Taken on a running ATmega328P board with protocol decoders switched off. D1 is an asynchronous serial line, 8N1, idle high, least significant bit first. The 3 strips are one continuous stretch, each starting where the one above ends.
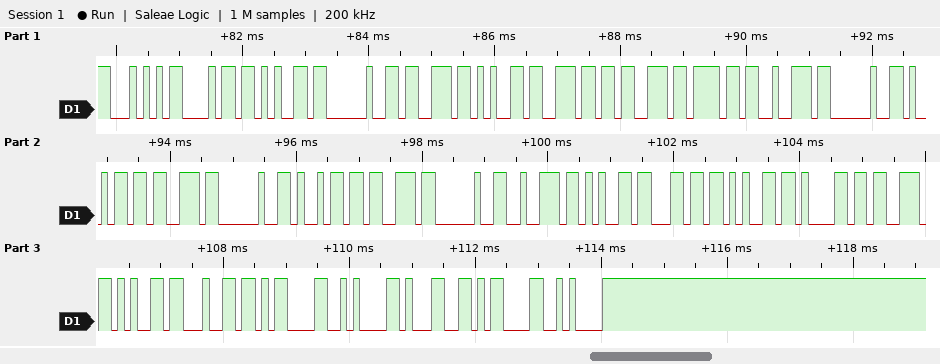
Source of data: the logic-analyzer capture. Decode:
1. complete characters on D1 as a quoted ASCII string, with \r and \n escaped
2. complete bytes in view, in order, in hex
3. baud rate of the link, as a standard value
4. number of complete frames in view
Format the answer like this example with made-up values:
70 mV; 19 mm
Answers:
"The sensor is is released\r\n1\r\n"; 54 68 65 20 73 65 6E 73 6F 72 20 69 73 20 69 73 20 72 65 6C 65 61 73 65 64 0D 0A 31 0D 0A; 9600 baud; 30
